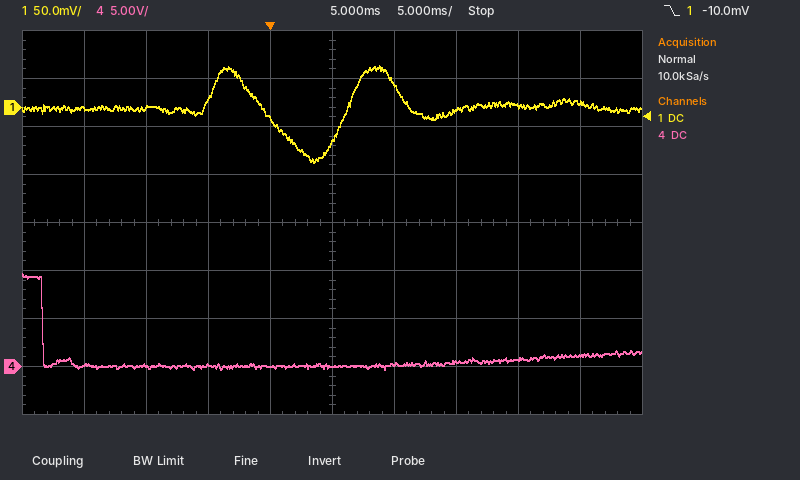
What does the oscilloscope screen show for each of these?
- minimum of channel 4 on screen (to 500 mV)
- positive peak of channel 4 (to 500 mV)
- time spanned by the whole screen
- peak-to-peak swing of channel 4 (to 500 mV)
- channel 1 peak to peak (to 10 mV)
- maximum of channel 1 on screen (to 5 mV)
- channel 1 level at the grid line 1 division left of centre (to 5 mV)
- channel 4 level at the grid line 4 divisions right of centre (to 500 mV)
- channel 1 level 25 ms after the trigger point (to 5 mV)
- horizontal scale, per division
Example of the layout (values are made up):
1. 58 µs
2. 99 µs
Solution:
1. -500 mV
2. 9.5 V
3. 50 ms
4. 10.0 V
5. 100 mV
6. 45 mV
7. -10 mV
8. 1.0 V
9. 5 mV
10. 5 ms
